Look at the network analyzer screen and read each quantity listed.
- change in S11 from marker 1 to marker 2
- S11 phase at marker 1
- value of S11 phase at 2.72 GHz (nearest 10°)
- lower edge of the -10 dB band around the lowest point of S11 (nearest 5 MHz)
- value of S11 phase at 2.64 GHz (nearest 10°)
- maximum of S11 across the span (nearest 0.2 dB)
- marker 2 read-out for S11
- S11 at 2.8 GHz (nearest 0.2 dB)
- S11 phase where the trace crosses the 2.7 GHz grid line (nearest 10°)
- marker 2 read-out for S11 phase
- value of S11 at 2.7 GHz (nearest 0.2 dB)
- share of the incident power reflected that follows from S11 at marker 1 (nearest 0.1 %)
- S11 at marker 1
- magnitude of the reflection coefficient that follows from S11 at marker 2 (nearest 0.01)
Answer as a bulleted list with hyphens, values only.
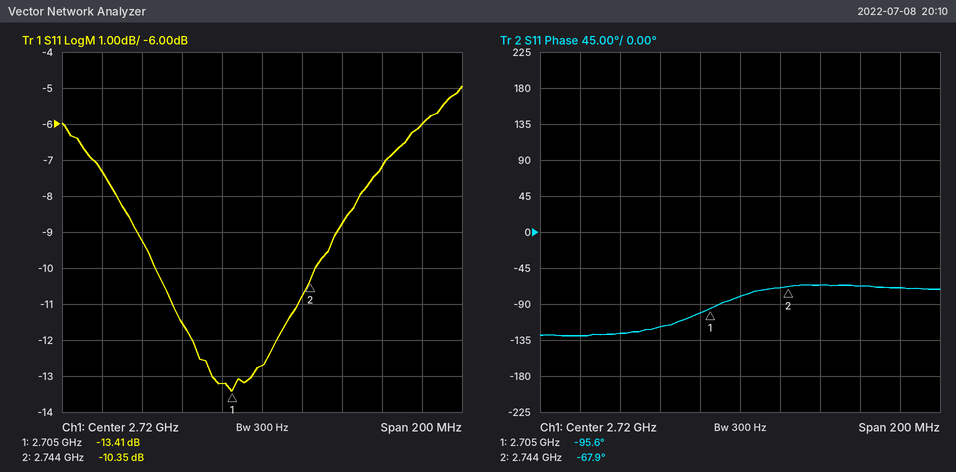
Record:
- 3.06 dB
- -95.6°
- -80°
- 2.665 GHz
- -130°
- -5.0 dB
- -10.35 dB
- -6.0 dB
- -100°
- -67.9°
- -13.2 dB
- 4.6 %
- -13.41 dB
- 0.30
